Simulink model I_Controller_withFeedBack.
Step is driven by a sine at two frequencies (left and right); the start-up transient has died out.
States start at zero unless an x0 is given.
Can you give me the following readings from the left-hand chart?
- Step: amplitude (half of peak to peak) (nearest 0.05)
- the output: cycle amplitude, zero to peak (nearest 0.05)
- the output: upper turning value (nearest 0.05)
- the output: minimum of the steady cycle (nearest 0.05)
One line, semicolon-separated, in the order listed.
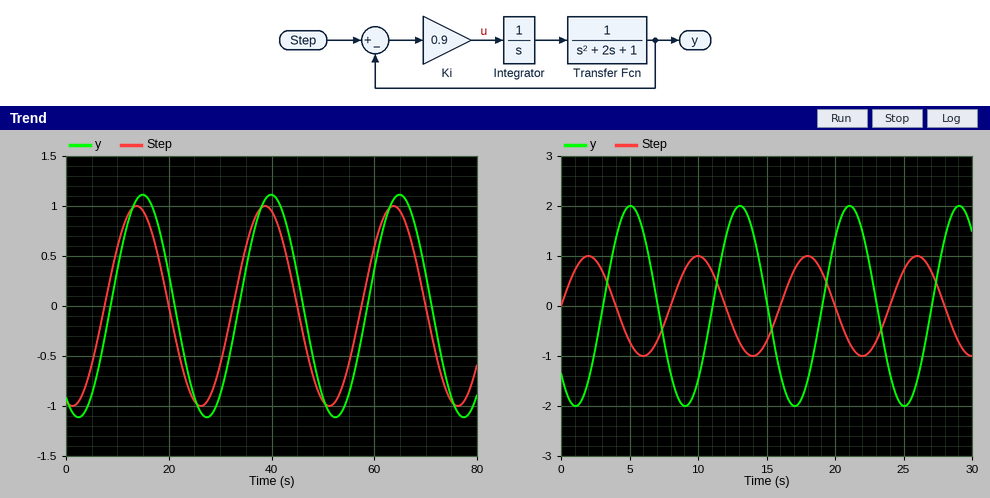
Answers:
1.00; 1.10; 1.10; -1.10
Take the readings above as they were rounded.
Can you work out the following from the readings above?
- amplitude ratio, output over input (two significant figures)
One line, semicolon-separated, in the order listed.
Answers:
1.1
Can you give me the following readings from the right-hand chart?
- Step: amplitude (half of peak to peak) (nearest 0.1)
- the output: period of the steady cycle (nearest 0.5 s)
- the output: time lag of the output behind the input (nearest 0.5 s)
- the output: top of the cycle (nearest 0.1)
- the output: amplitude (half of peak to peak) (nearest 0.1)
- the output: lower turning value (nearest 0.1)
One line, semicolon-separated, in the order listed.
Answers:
1.0; 8.0 s; 3.0 s; 2.0; 2.0; -2.0
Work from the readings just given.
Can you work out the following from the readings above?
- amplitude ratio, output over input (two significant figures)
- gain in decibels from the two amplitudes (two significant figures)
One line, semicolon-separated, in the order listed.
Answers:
2.0; 6.0 dB
